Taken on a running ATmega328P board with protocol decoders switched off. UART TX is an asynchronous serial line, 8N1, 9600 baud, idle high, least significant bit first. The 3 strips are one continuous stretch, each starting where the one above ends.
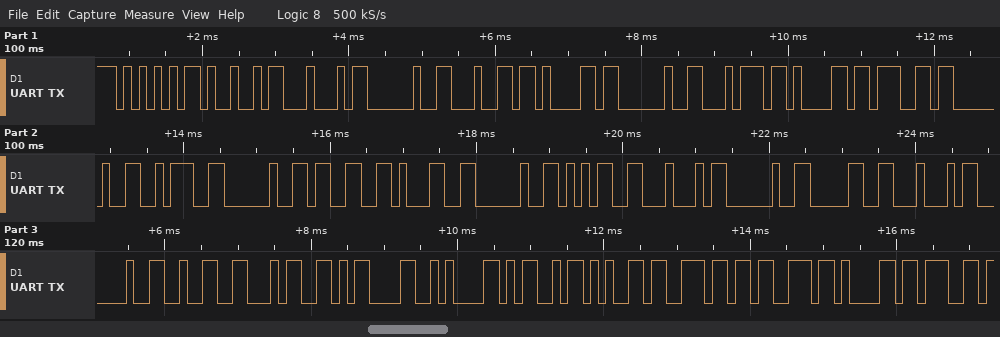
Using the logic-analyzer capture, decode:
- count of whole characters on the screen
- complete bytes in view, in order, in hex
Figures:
32
55 49 44 20 64 61 20 74 61 67 20 3A 20 33 31 20 35 44 20 30 44 20 32 34 0D 0A 4D 65 6E 73 61 67
